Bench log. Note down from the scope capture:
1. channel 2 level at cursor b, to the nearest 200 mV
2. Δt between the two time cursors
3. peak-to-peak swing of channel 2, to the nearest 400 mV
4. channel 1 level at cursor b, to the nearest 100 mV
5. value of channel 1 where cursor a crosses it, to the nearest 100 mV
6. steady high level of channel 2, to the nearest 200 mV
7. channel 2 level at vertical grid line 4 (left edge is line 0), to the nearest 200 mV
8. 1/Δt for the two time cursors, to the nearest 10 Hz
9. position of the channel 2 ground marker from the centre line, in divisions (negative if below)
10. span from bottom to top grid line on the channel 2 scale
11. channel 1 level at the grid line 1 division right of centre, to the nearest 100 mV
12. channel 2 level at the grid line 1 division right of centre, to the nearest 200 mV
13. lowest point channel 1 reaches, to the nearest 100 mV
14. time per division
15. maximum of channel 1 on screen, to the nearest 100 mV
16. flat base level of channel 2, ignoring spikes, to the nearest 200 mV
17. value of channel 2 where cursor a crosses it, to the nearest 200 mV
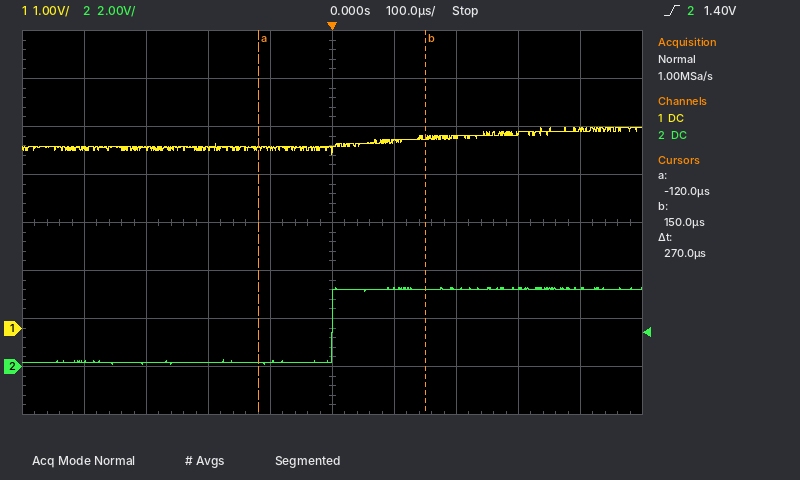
3.2 V
270 µs
3.2 V
4.0 V
3.7 V
3.2 V
200 mV
3.70 kHz
-3.0 div
16 V
3.9 V
3.2 V
3.6 V
100 µs
4.2 V
200 mV
200 mV
